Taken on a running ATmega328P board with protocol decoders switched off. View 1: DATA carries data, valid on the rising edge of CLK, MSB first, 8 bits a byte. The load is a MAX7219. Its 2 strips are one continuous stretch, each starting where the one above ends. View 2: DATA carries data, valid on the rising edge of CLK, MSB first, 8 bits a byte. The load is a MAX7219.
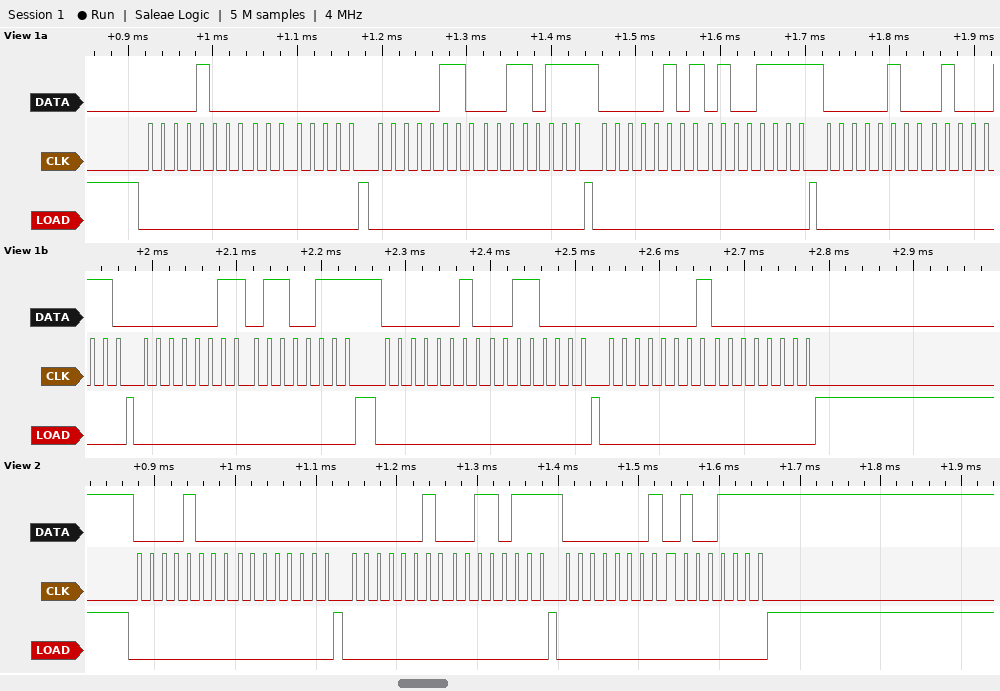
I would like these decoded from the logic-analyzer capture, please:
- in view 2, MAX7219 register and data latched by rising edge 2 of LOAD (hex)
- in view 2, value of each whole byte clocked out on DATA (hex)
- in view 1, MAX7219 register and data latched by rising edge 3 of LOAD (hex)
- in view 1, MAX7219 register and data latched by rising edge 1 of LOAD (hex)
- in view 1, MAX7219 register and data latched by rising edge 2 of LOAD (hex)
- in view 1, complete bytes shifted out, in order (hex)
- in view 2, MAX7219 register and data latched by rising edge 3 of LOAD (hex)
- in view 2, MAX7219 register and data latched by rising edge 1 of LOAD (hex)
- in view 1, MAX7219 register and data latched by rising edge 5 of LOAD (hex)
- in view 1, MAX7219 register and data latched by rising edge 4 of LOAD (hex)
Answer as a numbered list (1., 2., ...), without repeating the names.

1. register 0x2, data 0x37
2. 08 00 02 37 01 4F
3. register 0x5, data 0x4F
4. register 0x8, data 0x00
5. register 0x6, data 0x37
6. 08 00 06 37 05 4F 04 46 03 67 02 30 01 00
7. register 0x1, data 0x4F
8. register 0x8, data 0x00
9. register 0x3, data 0x67
10. register 0x4, data 0x46
